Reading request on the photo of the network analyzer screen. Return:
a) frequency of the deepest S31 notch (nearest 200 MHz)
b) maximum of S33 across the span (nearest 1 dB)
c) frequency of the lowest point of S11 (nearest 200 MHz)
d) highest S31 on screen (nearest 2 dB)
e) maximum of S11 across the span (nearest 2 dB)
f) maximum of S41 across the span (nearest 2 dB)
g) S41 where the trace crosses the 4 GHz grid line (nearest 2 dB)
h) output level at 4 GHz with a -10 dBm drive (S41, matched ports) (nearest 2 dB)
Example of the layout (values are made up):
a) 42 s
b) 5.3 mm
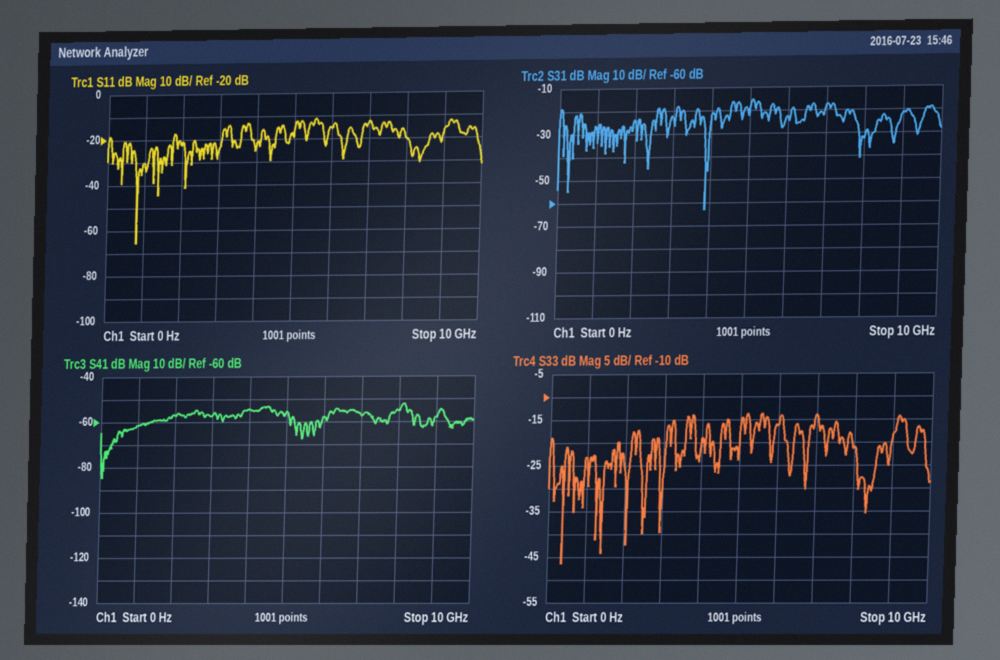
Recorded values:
a) 3.8 GHz
b) -14 dB
c) 800 MHz
d) -16 dB
e) -12 dB
f) -52 dB
g) -54 dB
h) -64 dBm
